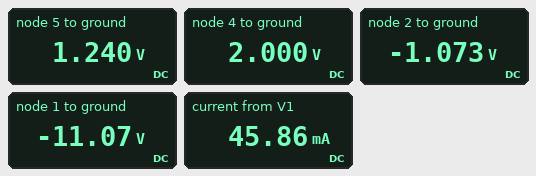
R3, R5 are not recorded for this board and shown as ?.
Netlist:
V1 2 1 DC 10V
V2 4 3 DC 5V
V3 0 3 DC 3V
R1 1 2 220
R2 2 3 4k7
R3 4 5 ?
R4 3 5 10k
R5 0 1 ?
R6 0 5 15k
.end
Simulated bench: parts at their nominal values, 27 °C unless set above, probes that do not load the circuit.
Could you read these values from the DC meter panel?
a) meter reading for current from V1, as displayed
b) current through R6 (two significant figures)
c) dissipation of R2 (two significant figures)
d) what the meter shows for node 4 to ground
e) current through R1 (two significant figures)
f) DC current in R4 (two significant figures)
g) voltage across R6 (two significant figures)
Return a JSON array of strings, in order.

["45.86 mA", "83 µA", "790 µW", "2.000 V", "45 mA", "420 µA", "1.2 V"]
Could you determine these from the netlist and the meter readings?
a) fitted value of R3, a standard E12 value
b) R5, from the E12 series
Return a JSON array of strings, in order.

["1.5 kΩ", "27 kΩ"]
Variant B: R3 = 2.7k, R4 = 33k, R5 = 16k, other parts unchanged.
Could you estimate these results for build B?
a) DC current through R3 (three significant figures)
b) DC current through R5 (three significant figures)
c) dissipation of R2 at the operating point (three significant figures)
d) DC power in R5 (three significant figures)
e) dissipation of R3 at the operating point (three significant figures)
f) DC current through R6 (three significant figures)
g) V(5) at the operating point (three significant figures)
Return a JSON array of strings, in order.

["226 µA", "628 µA", "1.85 mW", "6.31 mW", "138 µW", "92.7 µA", "1.39 V"]
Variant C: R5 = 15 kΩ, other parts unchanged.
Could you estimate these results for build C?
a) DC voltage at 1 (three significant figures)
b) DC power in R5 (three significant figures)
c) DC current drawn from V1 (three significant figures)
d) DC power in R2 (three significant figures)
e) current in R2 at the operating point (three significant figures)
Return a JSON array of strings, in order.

["-9.90 V", "6.53 mW", "46.1 mA", "2.05 mW", "660 µA"]
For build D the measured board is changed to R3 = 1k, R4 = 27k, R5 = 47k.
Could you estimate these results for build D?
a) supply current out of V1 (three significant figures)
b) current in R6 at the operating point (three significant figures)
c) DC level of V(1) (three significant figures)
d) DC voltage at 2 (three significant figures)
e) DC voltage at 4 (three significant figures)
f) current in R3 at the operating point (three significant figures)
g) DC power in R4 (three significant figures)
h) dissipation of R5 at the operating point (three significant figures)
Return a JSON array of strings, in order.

["45.7 mA", "114 µA", "-11.8 V", "-1.82 V", "2.00 V", "289 µA", "822 µW", "2.97 mW"]
